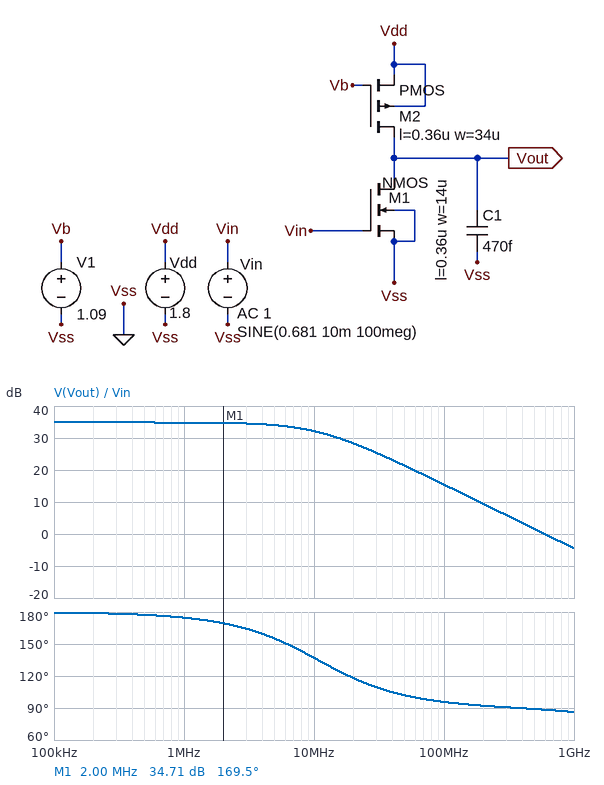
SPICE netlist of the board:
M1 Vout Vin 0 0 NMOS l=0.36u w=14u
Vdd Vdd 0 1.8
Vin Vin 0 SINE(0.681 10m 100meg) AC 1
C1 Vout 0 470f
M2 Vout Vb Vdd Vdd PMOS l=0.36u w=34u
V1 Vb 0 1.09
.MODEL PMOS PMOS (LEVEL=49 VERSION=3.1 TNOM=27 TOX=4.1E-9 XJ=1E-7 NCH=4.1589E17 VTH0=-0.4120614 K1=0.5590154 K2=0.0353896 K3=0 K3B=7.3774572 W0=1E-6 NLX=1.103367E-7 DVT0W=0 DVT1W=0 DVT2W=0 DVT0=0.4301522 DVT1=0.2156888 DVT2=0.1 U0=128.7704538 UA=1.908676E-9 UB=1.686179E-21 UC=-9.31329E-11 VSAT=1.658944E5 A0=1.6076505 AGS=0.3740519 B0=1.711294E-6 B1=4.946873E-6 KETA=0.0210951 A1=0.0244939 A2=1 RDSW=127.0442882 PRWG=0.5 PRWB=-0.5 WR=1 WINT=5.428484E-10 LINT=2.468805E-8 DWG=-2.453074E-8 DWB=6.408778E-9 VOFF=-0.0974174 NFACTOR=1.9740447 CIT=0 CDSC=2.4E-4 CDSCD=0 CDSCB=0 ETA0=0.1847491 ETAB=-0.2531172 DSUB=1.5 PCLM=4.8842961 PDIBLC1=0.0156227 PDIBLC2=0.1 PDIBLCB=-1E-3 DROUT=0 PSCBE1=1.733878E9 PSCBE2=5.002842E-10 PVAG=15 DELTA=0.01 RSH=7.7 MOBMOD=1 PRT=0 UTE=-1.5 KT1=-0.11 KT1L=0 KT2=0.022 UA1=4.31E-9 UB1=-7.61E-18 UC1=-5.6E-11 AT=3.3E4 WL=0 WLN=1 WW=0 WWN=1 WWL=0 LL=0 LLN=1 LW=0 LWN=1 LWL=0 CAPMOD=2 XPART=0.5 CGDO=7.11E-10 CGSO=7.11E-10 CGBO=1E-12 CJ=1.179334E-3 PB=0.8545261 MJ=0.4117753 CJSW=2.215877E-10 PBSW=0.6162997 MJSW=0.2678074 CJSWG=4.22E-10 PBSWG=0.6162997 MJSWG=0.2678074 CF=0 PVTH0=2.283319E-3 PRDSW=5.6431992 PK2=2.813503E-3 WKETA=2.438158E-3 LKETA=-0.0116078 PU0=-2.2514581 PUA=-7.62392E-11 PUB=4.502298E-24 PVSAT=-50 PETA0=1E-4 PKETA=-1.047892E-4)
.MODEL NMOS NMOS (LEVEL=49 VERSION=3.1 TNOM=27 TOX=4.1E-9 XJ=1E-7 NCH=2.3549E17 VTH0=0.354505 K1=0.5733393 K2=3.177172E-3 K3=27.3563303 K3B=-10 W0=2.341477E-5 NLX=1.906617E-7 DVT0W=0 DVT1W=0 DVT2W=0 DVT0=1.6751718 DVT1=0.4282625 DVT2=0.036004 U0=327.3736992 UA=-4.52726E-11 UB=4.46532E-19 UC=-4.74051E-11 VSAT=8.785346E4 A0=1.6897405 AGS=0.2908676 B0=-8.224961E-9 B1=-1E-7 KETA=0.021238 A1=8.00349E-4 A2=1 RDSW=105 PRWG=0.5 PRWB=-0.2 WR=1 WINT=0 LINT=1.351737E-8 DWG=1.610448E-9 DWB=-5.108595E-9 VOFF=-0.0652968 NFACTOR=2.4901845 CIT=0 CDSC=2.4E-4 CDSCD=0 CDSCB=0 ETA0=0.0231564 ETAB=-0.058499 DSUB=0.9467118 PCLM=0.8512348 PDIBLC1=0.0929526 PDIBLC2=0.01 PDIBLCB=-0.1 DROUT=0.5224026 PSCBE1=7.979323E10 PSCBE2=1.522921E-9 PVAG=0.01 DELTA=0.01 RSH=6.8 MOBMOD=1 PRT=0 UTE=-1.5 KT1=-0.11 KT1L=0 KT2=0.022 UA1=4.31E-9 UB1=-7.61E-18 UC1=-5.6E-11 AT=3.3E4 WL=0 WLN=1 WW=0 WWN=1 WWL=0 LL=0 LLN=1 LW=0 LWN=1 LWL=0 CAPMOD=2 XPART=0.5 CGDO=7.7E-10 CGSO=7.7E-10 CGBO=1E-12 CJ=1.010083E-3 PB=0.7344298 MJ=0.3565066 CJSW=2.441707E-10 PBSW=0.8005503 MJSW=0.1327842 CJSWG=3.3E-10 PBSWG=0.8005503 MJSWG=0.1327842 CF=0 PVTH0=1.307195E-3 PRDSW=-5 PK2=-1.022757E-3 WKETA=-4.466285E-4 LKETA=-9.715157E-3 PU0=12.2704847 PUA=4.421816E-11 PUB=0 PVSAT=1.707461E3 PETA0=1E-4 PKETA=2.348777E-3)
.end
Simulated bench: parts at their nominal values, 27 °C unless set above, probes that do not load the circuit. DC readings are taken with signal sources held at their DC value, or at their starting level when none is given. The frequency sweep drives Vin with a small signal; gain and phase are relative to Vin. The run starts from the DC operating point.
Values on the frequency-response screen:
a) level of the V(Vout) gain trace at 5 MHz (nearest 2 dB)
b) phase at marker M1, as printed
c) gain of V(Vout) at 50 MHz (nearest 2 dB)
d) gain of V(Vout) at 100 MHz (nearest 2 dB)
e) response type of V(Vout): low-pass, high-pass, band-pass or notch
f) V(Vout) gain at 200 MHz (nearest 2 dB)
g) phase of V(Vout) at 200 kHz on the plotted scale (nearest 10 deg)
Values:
34 dB
169.5 deg
22 dB
16 dB
low-pass
10 dB
180 deg
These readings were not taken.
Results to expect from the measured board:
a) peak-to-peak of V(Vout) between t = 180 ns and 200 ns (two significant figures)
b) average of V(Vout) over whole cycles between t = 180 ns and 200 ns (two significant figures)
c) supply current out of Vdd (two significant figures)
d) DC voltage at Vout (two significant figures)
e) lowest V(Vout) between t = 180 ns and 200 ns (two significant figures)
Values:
120 mV
900 mV
190 µA
900 mV
840 mV
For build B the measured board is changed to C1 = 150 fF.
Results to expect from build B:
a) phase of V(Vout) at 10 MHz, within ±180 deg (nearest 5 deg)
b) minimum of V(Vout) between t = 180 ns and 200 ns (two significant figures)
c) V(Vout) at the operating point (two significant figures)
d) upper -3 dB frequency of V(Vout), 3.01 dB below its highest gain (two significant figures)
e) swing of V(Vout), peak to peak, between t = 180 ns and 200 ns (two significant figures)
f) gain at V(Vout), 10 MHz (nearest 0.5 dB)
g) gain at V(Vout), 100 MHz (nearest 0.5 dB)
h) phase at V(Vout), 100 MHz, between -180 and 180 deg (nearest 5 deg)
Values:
160 deg
750 mV
900 mV
28 MHz
300 mV
34.5 dB
23.5 dB
105 deg
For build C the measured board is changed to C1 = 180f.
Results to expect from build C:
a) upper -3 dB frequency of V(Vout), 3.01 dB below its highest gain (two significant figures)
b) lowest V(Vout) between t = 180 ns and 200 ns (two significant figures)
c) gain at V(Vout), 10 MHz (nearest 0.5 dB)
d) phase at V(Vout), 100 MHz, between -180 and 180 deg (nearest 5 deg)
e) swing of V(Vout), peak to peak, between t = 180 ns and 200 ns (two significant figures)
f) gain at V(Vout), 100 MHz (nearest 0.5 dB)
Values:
24 MHz
770 mV
34.0 dB
105 deg
260 mV
22.5 dB
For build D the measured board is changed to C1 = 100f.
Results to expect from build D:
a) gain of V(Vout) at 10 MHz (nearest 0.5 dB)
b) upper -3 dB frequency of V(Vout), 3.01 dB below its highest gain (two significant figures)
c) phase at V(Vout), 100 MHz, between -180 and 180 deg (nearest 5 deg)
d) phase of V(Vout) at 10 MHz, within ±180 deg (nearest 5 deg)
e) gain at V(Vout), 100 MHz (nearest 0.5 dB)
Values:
34.5 dB
37 MHz
110 deg
165 deg
25.5 dB
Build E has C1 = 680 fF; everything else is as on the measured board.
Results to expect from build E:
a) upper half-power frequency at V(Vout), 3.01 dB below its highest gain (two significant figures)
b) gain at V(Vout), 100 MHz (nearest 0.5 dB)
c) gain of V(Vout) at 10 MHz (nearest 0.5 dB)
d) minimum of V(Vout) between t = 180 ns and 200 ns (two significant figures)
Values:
7.7 MHz
12.5 dB
30.5 dB
850 mV
